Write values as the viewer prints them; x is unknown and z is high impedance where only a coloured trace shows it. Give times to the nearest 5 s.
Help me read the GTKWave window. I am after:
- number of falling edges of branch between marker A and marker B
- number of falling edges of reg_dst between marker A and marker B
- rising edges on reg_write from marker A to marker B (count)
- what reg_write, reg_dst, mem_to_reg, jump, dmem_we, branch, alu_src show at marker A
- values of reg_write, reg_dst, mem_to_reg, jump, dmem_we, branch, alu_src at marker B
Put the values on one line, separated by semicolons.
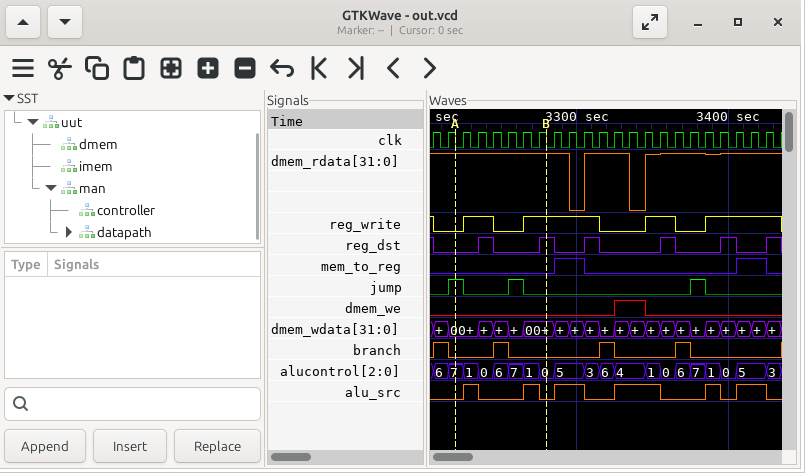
1; 1; 2; reg_write=0, reg_dst=0, mem_to_reg=0, jump=1, dmem_we=0, branch=0, alu_src=0; reg_write=1, reg_dst=1, mem_to_reg=0, jump=0, dmem_we=0, branch=0, alu_src=0
